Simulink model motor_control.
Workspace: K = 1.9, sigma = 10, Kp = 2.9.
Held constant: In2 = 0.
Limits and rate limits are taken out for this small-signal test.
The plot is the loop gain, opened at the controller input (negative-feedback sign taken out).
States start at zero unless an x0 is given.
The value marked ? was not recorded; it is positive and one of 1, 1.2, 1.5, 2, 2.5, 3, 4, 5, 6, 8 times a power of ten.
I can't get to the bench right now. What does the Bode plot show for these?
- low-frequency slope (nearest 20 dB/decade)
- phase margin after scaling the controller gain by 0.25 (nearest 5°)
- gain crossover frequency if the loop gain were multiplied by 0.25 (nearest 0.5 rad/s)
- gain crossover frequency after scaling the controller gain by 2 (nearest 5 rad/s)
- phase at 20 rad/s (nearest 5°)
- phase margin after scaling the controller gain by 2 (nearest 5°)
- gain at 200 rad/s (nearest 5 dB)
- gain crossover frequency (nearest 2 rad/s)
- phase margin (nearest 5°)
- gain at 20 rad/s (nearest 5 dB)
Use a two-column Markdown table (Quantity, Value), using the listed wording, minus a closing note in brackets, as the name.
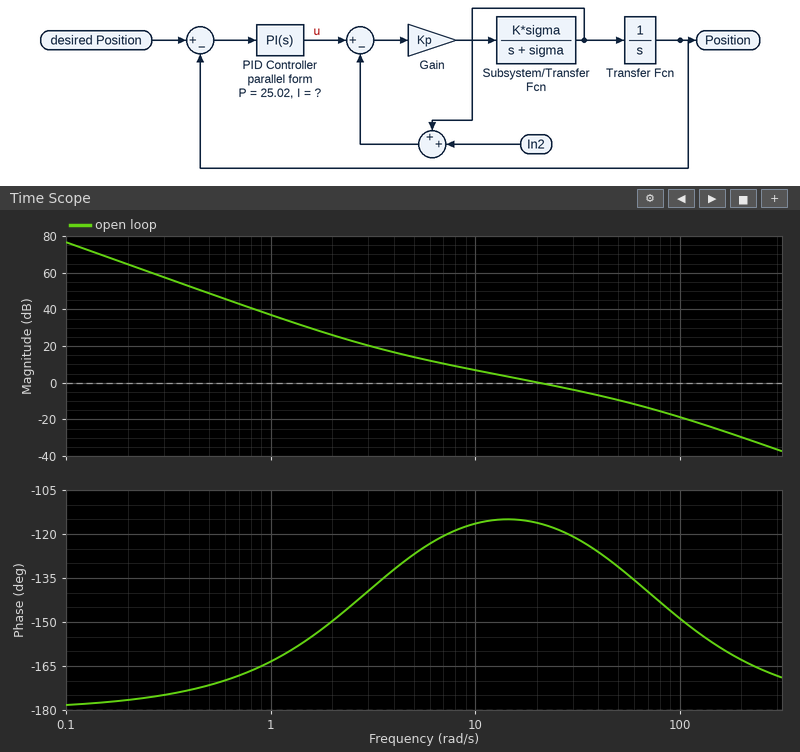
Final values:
| Quantity | Value |
|---|---|
| low-frequency slope | -40 dB/decade |
| phase margin after scaling the controller gain by 0.25 | 55° |
| gain crossover frequency if the loop gain were multiplied by 0.25 | 6.0 rad/s |
| gain crossover frequency after scaling the controller gain by 2 | 35 rad/s |
| phase at 20 rad/s | -115° |
| phase margin after scaling the controller gain by 2 | 55° |
| gain at 200 rad/s | -30 dB |
| gain crossover frequency | 20 rad/s |
| phase margin | 65° |
| gain at 20 rad/s | 0 dB |
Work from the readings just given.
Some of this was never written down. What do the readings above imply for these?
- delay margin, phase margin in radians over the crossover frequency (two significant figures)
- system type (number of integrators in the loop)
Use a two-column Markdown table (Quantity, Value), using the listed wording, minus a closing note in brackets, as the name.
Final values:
| Quantity | Value |
|---|---|
| delay margin, phase margin in radians over the crossover frequency | 0.057 s |
| system type | 2 |
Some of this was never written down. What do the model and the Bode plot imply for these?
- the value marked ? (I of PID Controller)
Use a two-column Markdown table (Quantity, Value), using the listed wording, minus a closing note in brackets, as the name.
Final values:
| Quantity | Value |
|---|---|
| the value marked ? | 80 |
